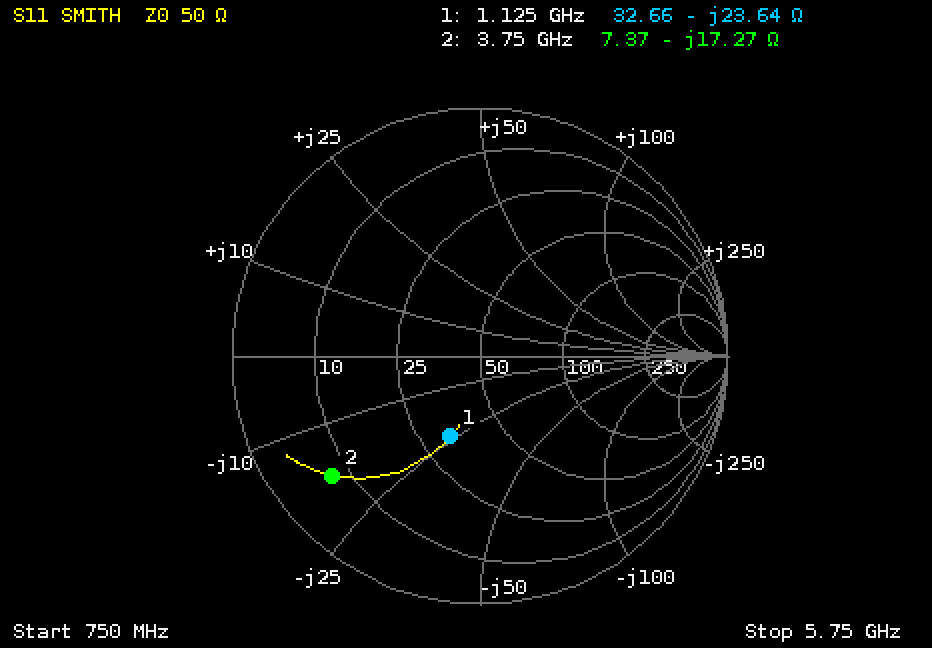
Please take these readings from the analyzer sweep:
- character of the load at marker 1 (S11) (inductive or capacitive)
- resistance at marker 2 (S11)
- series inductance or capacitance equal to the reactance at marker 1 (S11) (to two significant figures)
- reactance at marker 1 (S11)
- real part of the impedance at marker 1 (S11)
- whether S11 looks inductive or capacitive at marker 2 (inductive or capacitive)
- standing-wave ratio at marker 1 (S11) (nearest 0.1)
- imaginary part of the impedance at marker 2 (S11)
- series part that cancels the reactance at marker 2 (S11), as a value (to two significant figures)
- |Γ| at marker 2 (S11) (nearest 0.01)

capacitive
7.37 Ω
6.0 pF
-23.64 Ω
32.66 Ω
capacitive
2.0
-17.27 Ω
730 pH
0.77
